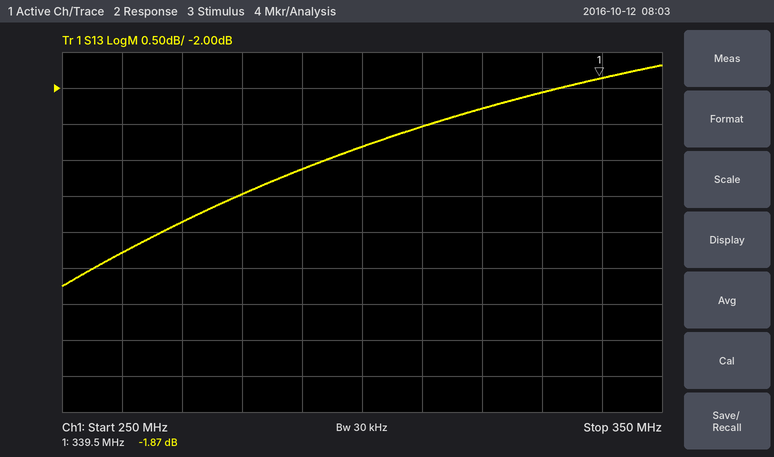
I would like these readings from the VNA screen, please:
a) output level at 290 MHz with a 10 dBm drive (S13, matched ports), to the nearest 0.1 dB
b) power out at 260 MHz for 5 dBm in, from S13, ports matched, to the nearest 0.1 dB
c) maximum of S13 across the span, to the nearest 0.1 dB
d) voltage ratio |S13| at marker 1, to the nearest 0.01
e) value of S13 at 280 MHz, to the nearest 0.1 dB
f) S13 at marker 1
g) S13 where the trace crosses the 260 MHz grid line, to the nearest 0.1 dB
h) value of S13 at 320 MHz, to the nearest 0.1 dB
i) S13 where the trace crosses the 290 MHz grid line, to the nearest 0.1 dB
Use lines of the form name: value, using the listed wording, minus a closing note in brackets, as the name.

output level at 290 MHz with a 10 dBm drive (S13, matched ports), to the nearest 0.1 dB: 6.9 dBm
power out at 260 MHz for 5 dBm in, from S13, ports matched, to the nearest 0.1 dB: 0.7 dBm
maximum of S13 across the span, to the nearest 0.1 dB: -1.7 dB
voltage ratio |S13| at marker 1, to the nearest 0.01: 0.81
value of S13 at 280 MHz, to the nearest 0.1 dB: -3.5 dB
S13 at marker 1: -1.87 dB
S13 where the trace crosses the 260 MHz grid line, to the nearest 0.1 dB: -4.3 dB
value of S13 at 320 MHz, to the nearest 0.1 dB: -2.3 dB
S13 where the trace crosses the 290 MHz grid line, to the nearest 0.1 dB: -3.1 dB
